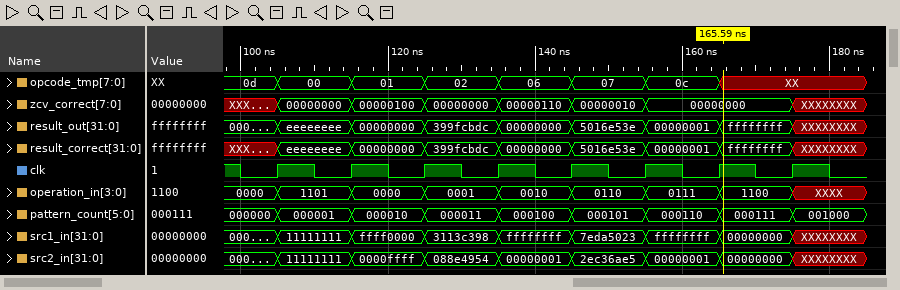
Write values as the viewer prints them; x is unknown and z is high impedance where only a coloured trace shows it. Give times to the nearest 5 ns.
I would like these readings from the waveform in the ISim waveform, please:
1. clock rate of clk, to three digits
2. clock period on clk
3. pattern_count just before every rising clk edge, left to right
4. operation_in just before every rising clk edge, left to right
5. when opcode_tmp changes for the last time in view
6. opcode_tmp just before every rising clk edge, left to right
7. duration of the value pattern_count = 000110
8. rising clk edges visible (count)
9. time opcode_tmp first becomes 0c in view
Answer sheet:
100 MHz
10 ns
000000, 000001, 000010, 000011, 000100, 000101, 000110, 000111
0000, 1101, 0000, 0001, 0010, 0110, 0111, 1100
165 ns
0d, 00, 01, 02, 06, 07, 0c, XX
10 ns
8
155 ns
